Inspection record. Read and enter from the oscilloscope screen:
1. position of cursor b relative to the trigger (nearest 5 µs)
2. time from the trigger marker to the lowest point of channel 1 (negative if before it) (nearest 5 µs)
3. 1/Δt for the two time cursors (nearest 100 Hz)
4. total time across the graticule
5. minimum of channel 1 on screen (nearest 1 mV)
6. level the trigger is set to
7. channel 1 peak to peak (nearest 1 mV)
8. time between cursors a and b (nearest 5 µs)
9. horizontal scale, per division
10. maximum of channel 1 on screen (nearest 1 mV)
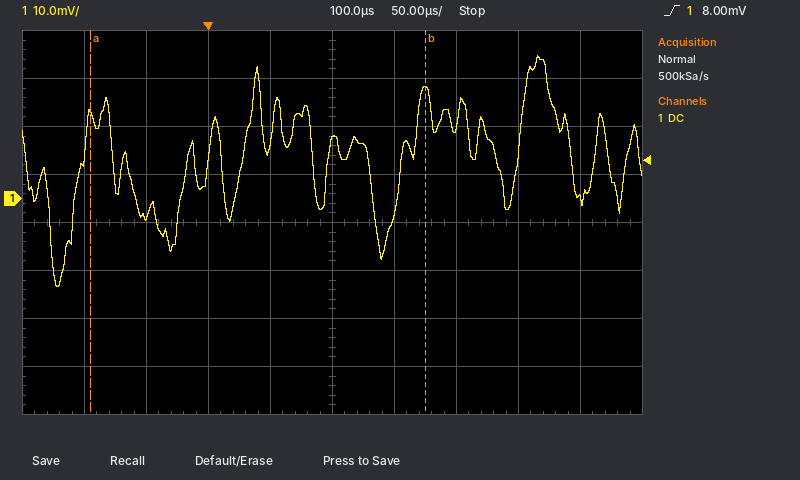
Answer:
+175 µs
-120 µs
3.7 kHz
500 µs
-18 mV
8.00 mV
48 mV
270 µs
50 µs
30 mV
